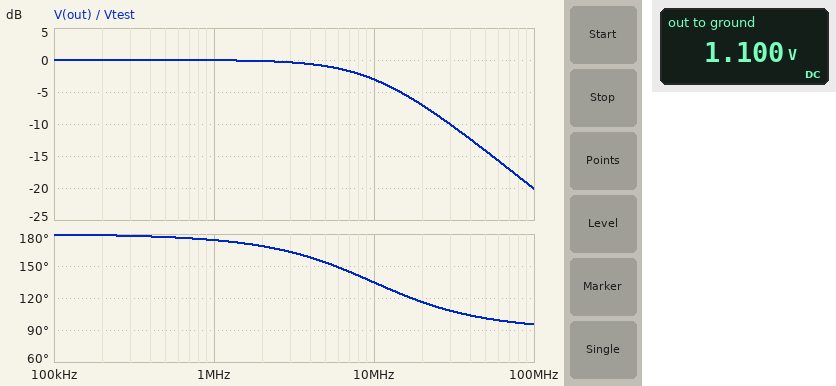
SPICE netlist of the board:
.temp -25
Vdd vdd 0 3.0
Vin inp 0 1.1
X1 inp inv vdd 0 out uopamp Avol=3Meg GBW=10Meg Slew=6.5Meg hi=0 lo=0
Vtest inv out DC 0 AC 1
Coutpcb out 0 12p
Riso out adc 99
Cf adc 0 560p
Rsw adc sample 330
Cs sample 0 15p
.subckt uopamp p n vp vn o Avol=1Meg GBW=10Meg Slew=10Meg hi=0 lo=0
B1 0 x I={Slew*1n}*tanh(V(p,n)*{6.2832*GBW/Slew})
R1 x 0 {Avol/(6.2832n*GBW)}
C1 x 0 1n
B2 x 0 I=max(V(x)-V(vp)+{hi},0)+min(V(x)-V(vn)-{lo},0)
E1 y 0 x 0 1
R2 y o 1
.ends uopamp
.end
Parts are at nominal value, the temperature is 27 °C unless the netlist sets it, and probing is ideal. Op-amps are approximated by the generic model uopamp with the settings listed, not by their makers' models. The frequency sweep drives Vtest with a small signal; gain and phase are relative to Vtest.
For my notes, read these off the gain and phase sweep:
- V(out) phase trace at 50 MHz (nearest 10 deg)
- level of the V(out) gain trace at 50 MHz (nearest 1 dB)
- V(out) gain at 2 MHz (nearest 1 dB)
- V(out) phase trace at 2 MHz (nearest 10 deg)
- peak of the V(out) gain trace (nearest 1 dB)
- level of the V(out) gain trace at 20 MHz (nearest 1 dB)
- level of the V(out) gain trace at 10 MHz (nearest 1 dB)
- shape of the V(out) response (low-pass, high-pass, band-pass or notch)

100 deg
-14 dB
0 dB
170 deg
0 dB
-7 dB
-3 dB
low-pass
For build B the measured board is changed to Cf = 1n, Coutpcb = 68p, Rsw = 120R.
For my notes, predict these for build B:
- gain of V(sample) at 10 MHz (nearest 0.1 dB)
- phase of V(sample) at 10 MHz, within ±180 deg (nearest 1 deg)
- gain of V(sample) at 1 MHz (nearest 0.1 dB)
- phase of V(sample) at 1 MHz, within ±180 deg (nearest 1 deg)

-19.2 dB
47 deg
-1.5 dB
141 deg
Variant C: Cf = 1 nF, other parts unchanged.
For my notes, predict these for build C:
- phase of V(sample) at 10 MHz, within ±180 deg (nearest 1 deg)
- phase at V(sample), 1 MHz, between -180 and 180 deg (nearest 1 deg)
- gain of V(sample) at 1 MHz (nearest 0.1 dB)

37 deg
140 deg
-1.5 dB
